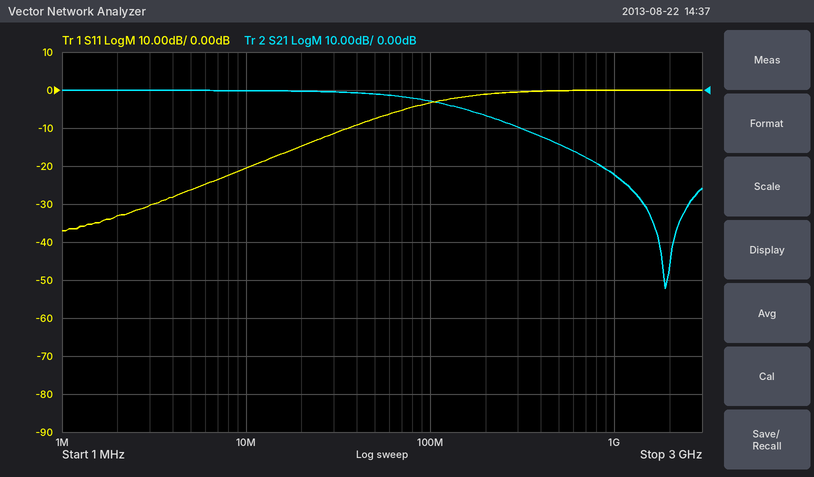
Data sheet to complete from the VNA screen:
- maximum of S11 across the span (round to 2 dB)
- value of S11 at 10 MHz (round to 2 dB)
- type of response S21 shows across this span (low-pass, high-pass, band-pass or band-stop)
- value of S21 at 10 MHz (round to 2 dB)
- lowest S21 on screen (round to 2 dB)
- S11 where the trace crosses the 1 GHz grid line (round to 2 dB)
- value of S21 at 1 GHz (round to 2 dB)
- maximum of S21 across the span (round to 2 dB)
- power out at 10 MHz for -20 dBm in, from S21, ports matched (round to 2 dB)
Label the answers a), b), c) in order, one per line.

a) 0 dB
b) -20 dB
c) low-pass
d) 0 dB
e) -52 dB
f) 0 dB
g) -22 dB
h) 0 dB
i) -20 dBm
